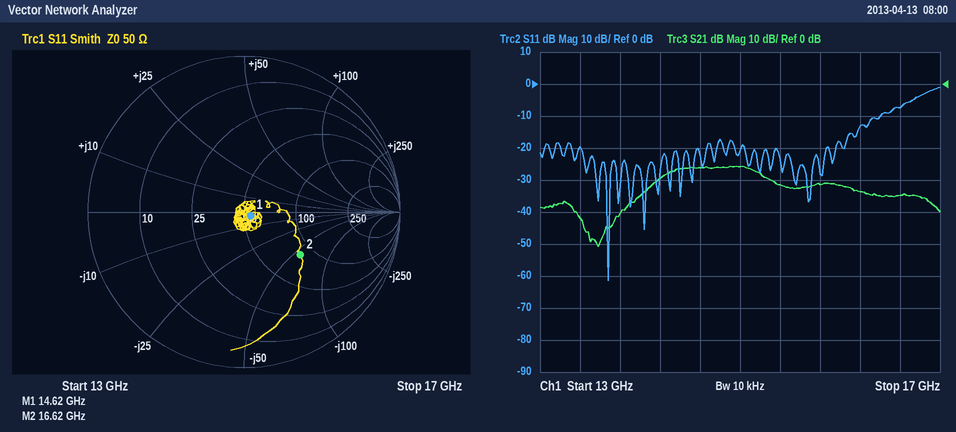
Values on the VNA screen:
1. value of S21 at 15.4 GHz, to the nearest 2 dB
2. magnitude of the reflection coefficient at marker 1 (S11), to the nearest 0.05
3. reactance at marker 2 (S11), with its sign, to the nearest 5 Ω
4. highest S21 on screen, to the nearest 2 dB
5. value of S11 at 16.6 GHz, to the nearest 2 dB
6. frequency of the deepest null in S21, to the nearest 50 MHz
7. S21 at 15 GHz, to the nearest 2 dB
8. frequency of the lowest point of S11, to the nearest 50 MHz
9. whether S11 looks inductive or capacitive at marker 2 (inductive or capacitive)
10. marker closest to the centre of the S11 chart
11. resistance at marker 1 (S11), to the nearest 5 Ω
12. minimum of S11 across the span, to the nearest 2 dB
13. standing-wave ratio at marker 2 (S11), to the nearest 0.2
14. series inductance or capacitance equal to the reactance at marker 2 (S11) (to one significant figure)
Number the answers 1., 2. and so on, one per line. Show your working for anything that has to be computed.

1. -32 dB
2. 0.05
3. -55 Ω
4. -26 dB
5. -8 dB
6. 13.60 GHz
7. -26 dB
8. 13.70 GHz
9. capacitive
10. marker 1
11. 55 Ω
12. -62 dB
13. 2.6
14. C = 1/(2π × 16.62 GHz × 55 Ω) ≈ 174 fF, so 200 fF to one significant figure
